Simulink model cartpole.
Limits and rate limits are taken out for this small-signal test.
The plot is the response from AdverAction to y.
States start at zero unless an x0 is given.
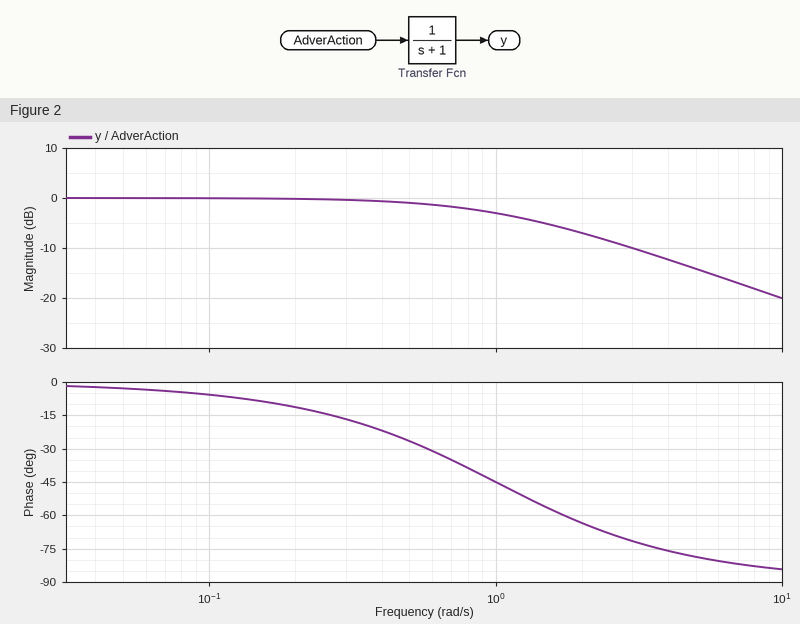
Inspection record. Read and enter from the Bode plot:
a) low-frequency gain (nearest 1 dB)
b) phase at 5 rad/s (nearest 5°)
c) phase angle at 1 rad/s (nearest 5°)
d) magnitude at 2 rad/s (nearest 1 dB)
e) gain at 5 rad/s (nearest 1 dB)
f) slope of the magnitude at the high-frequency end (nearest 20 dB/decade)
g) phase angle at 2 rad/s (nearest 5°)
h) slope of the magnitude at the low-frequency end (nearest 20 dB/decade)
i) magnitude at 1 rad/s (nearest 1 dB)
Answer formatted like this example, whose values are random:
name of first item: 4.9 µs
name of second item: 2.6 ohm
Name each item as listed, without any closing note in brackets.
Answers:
low-frequency gain: 0 dB
phase at 5 rad/s: -80°
phase angle at 1 rad/s: -45°
magnitude at 2 rad/s: -7 dB
gain at 5 rad/s: -14 dB
slope of the magnitude at the high-frequency end: -20 dB/decade
phase angle at 2 rad/s: -65°
slope of the magnitude at the low-frequency end: 0 dB/decade
magnitude at 1 rad/s: -3 dB
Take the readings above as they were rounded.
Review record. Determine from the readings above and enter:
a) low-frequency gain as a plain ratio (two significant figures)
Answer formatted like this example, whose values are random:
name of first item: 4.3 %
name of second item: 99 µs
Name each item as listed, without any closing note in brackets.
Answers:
low-frequency gain as a plain ratio: 1.0
